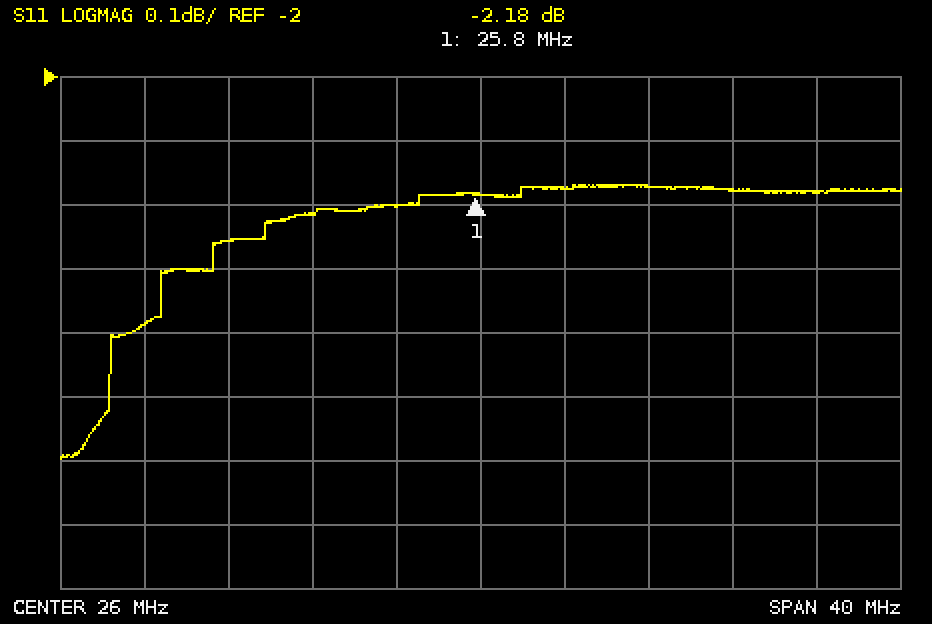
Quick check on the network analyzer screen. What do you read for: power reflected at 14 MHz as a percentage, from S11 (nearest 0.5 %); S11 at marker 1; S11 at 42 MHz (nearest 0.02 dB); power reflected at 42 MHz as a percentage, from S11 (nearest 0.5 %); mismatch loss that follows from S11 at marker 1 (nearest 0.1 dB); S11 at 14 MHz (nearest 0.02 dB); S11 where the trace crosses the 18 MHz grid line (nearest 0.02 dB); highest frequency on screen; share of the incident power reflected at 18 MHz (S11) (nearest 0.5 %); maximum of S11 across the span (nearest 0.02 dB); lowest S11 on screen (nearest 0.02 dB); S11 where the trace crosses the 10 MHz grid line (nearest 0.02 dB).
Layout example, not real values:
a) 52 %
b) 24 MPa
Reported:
a) 59.5 %
b) -2.18 dB
c) -2.18 dB
d) 60.5 %
e) 4.0 dB
f) -2.26 dB
g) -2.22 dB
h) 46 MHz
i) 60.0 %
j) -2.16 dB
k) -2.60 dB
l) -2.38 dB
